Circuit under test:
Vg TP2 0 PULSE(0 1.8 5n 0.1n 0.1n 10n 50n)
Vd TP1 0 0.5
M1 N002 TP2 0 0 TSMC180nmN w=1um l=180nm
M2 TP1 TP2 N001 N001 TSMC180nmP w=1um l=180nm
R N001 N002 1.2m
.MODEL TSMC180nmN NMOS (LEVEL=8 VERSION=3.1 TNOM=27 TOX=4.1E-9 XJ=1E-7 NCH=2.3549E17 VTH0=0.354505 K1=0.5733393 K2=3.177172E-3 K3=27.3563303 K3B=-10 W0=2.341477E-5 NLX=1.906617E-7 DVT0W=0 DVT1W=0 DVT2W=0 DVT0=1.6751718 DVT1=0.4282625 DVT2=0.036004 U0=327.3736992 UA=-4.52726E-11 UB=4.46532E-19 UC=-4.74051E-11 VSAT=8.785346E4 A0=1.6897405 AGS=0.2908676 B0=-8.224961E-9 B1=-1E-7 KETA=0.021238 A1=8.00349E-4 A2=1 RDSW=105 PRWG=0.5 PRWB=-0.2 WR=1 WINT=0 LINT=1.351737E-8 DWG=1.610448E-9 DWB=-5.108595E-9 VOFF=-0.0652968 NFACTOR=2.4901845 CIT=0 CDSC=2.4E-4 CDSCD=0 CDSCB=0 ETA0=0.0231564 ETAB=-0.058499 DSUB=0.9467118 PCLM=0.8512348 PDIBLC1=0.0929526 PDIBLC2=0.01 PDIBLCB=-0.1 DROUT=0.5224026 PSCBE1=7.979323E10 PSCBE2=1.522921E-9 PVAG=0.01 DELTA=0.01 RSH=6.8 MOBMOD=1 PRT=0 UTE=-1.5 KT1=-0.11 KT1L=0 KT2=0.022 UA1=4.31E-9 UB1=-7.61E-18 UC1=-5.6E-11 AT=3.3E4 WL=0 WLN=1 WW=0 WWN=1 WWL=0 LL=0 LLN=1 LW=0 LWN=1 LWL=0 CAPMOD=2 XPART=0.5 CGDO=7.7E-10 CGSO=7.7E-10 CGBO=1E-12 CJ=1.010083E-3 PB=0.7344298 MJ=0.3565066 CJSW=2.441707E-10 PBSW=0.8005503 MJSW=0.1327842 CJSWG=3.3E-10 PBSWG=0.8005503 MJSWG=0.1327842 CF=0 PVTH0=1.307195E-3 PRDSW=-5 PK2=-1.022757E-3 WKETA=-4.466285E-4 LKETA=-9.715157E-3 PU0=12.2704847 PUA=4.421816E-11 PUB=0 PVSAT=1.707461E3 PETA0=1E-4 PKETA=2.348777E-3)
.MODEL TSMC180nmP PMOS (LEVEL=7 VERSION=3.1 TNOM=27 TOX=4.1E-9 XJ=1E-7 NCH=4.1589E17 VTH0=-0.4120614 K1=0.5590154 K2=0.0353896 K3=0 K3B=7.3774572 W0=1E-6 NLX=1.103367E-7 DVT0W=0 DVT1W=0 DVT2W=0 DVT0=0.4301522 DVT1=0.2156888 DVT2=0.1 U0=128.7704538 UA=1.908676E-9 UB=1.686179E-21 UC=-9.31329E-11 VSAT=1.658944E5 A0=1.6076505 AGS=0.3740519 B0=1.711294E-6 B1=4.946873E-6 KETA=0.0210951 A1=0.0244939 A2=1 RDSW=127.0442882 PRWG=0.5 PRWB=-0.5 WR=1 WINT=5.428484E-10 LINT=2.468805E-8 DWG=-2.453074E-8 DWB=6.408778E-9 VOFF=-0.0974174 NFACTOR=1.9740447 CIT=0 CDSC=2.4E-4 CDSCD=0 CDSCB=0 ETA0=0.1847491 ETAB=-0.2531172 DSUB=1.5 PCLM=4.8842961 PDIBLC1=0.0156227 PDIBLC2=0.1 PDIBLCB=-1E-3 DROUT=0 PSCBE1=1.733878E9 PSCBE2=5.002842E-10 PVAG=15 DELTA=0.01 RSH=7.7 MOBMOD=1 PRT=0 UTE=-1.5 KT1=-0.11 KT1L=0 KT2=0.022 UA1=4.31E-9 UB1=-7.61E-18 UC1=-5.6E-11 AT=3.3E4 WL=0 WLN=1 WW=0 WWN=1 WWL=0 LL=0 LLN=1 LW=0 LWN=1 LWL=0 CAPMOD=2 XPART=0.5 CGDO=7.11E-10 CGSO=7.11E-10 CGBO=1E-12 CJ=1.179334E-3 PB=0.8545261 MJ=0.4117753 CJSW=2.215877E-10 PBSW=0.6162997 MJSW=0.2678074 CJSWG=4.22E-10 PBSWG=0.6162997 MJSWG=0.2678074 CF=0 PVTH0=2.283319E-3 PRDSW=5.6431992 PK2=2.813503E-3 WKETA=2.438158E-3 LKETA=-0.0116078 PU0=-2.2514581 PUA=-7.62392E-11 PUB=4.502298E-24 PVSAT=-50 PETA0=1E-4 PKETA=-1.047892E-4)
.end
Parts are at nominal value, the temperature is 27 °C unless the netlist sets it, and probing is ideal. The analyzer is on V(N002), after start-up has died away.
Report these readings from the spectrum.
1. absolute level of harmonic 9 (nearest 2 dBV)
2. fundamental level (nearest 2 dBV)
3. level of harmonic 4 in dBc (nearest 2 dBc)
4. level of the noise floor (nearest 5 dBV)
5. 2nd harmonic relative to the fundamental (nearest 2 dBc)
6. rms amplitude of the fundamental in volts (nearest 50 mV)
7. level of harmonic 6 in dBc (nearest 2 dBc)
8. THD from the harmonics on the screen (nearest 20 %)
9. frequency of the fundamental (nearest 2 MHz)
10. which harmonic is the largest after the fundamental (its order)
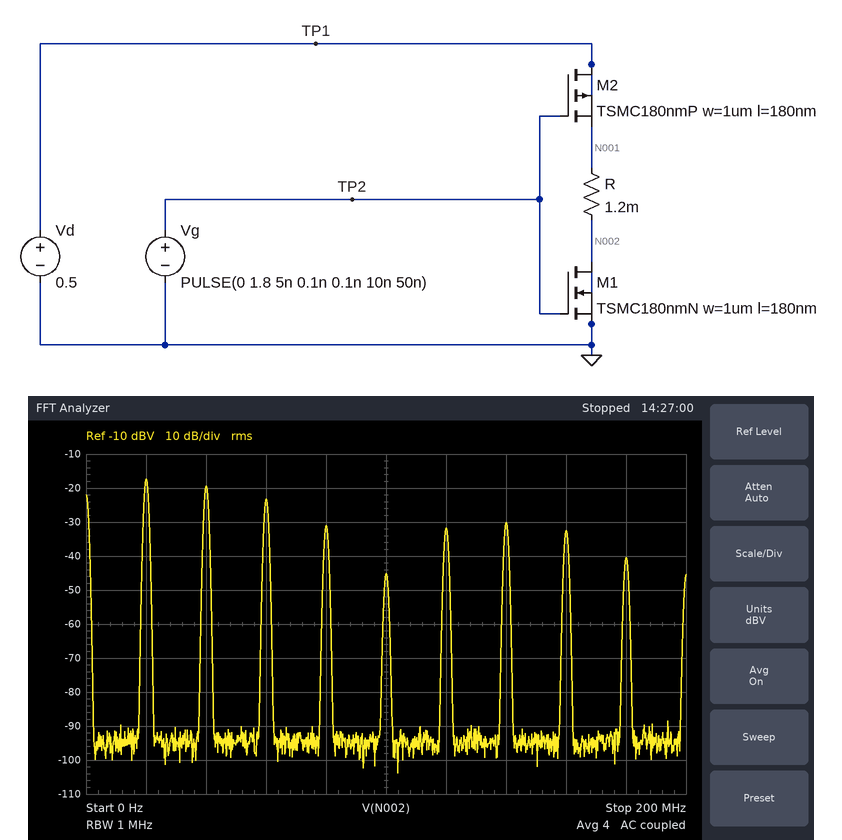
-40 dBV
-18 dBV
-14 dBc
-95 dBV
-2 dBc
150 mV
-14 dBc
100 %
20 MHz
2
